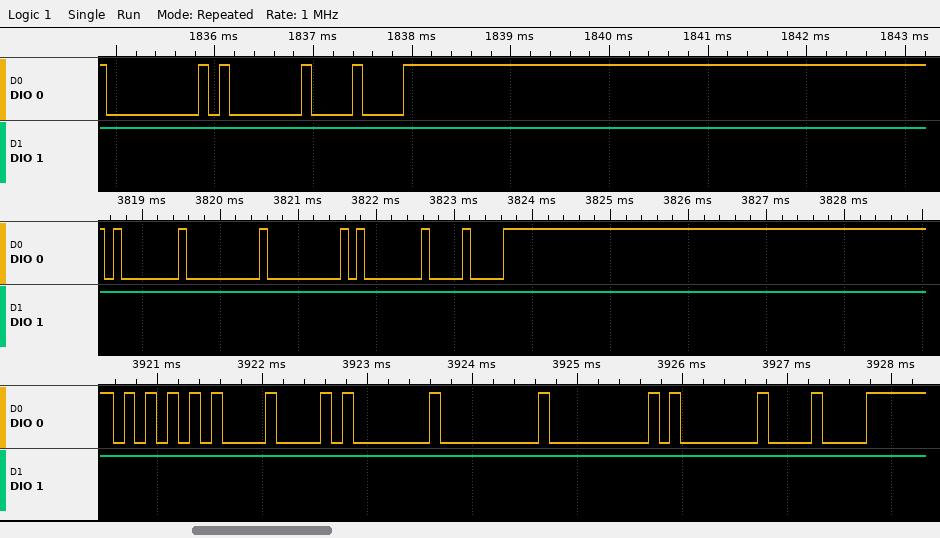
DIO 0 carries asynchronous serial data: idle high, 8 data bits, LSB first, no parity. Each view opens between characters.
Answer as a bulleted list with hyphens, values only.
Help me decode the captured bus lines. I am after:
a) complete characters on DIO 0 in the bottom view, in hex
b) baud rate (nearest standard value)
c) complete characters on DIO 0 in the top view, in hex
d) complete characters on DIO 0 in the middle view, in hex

- 55, 08, 01, 00, 00, 01, 08
- 9600 baud
- 00, 01, 08
- 01, 00, 00, 01, 08
